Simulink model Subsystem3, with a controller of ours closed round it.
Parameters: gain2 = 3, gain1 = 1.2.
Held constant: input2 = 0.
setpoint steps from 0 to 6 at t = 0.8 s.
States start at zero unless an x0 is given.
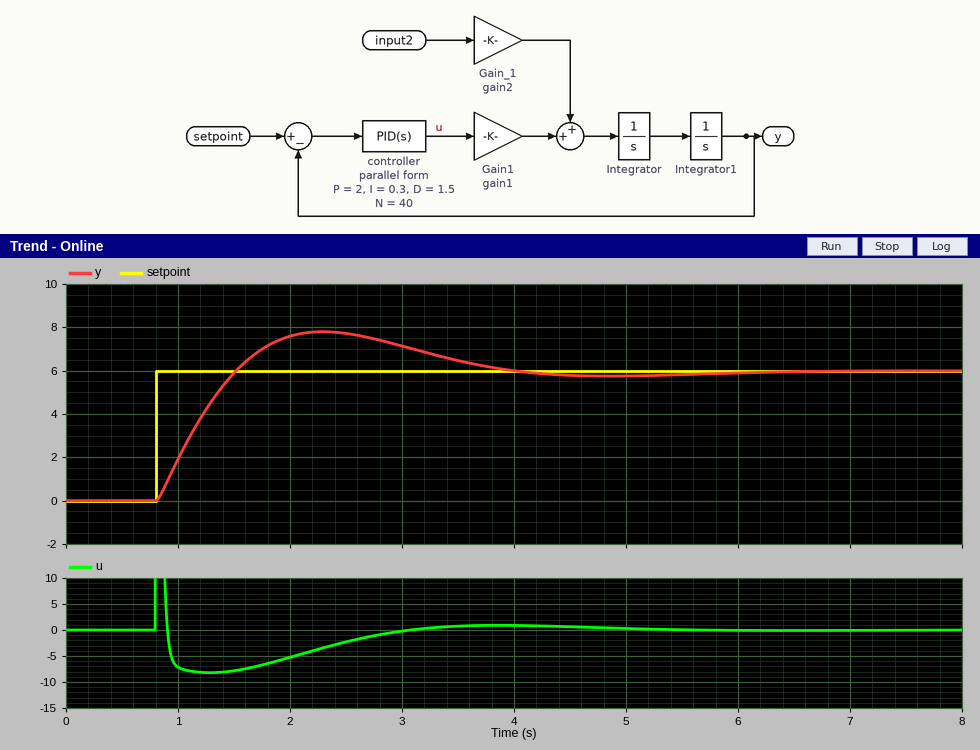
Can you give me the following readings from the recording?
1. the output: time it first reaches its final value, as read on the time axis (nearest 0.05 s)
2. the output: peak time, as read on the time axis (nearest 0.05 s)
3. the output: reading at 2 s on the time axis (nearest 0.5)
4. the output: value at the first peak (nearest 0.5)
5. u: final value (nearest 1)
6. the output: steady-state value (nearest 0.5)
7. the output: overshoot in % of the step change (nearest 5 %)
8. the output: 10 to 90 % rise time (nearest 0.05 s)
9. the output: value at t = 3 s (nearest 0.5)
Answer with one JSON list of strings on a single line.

["1.50 s", "2.30 s", "7.5", "8.0", "0", "6.0", "30 %", "0.55 s", "7.0"]
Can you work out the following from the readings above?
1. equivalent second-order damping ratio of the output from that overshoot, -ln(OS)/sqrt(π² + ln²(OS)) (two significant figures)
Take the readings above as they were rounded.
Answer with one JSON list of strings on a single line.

["0.36"]
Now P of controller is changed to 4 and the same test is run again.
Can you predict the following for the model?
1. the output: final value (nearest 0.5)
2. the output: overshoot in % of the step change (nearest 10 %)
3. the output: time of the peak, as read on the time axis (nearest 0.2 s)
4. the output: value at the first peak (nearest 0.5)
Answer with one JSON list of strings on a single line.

["6.0", "40 %", "2.0 s", "8.5"]
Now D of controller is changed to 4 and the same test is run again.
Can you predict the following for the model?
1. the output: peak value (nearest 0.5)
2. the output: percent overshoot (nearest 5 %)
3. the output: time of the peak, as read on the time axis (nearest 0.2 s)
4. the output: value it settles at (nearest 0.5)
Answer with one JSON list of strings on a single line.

["6.5", "10 %", "1.8 s", "6.0"]
